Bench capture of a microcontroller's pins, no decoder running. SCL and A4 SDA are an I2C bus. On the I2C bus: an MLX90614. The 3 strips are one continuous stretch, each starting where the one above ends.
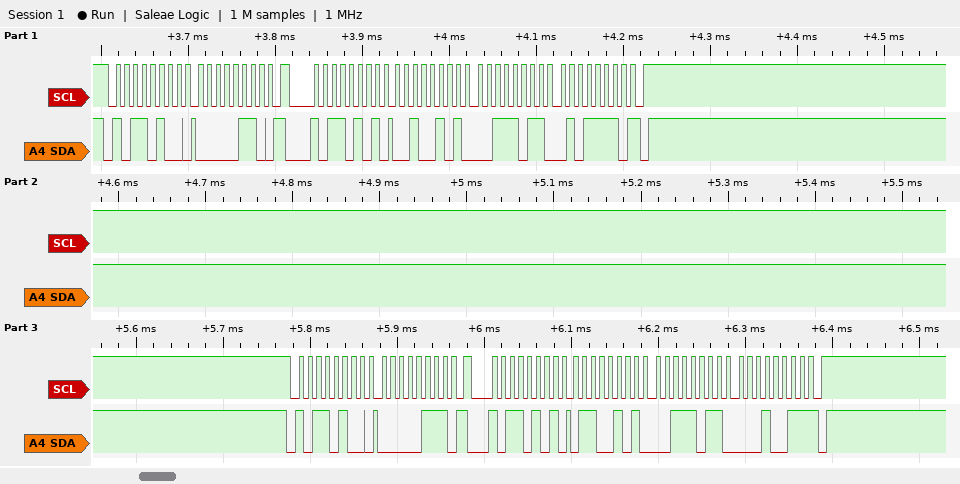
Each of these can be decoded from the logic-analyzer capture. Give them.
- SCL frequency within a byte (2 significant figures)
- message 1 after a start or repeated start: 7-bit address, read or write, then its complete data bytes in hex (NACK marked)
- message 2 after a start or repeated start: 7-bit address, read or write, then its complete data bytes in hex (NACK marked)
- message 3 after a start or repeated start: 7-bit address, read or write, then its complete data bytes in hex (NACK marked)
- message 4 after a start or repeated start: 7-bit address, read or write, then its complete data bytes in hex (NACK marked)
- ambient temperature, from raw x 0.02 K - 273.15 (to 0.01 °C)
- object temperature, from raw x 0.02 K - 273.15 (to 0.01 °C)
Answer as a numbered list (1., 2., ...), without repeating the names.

1. 100 kHz
2. 0x5A write: 06
3. 0x5A read: 25 3B 5E NACK
4. 0x5A write: 07
5. 0x5A read: 65 3B 13 NACK
6. 29.67 °C
7. 30.95 °C
